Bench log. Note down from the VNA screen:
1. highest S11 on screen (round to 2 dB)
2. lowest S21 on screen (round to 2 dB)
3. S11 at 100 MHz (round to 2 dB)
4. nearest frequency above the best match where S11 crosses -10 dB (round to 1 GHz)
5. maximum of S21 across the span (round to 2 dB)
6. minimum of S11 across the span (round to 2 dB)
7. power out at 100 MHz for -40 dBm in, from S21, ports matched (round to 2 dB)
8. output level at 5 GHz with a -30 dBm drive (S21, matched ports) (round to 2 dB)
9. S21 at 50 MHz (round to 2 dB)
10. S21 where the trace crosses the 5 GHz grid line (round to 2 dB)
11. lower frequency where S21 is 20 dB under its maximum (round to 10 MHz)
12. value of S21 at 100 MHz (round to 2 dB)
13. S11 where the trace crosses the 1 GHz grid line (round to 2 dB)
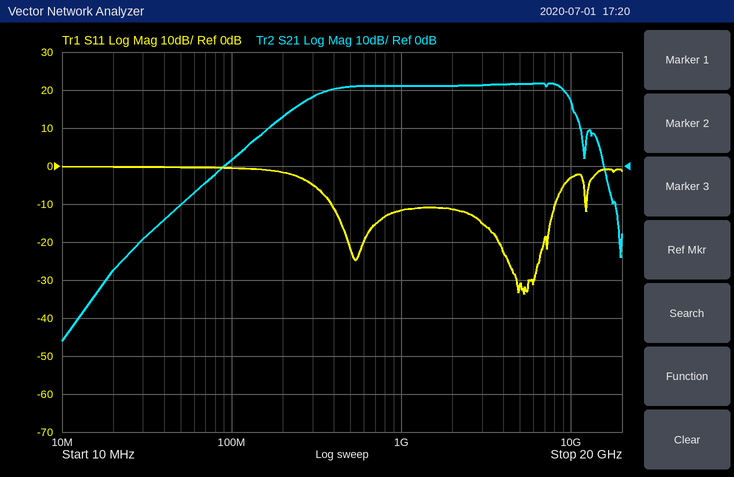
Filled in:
0 dB
-46 dB
0 dB
8 GHz
22 dB
-34 dB
-38 dBm
-8 dBm
-10 dB
22 dB
100 MHz
2 dB
-12 dB
